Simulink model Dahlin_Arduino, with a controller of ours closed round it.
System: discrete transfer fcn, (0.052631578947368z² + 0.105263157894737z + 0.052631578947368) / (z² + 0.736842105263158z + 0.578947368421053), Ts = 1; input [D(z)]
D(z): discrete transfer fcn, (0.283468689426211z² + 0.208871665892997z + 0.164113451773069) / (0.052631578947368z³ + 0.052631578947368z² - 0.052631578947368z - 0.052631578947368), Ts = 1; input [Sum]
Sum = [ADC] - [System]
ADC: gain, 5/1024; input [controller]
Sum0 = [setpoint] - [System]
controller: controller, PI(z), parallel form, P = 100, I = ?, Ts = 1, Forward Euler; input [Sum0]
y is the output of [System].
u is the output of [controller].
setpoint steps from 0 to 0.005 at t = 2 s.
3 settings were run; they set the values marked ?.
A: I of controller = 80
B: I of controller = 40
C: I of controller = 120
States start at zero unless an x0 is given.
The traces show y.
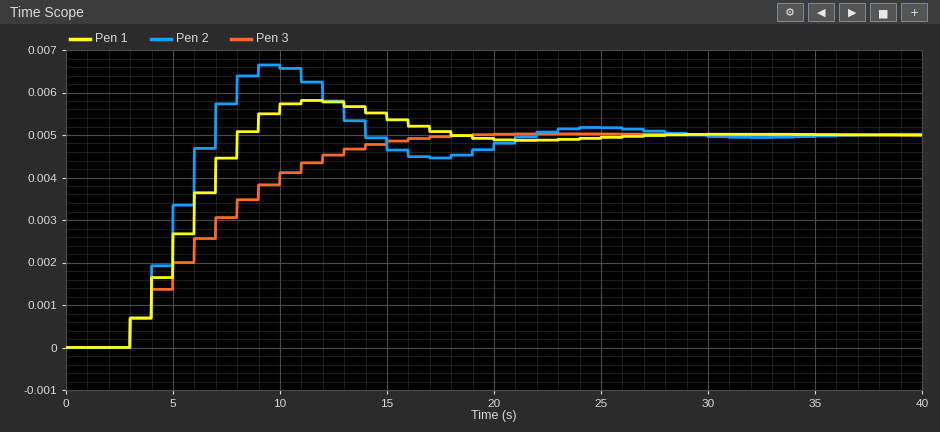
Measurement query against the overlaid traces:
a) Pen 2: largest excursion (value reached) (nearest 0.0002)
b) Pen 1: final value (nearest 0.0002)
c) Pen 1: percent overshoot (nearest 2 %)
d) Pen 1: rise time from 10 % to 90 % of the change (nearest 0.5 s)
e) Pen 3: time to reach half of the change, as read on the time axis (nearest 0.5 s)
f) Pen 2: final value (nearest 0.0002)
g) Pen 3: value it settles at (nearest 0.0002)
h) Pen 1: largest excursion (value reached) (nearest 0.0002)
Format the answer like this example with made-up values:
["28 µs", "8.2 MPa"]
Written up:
["0.0066", "0.0050", "16 %", "5.0 s", "6.0 s", "0.0050", "0.0050", "0.0058"]
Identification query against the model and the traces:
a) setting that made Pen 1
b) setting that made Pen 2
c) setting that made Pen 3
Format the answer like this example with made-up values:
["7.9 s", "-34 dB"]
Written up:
["A", "C", "B"]
